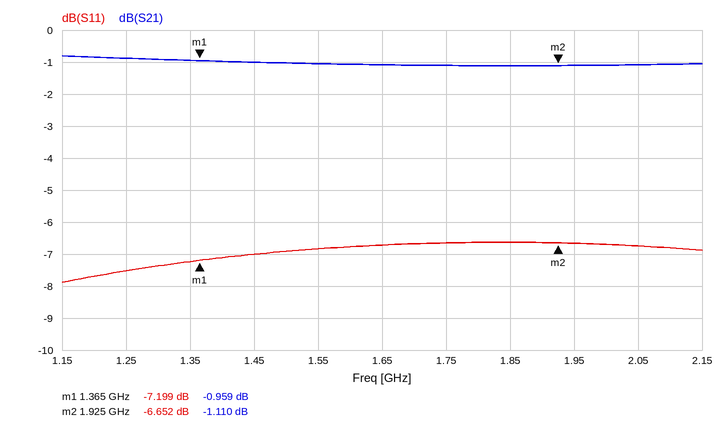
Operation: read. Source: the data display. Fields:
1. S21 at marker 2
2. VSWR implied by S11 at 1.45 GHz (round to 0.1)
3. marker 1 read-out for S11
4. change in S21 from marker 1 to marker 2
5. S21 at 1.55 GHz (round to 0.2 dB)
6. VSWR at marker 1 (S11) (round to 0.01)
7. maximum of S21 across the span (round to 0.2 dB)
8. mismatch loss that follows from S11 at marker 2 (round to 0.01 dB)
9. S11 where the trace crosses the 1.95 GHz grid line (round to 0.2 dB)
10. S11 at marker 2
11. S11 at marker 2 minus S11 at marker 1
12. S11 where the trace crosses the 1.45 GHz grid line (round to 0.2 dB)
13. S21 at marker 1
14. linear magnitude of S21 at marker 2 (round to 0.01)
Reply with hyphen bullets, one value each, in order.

- -1.110 dB
- 2.6
- -7.199 dB
- -0.151 dB
- -1.0 dB
- 2.55
- -0.8 dB
- 1.06 dB
- -6.6 dB
- -6.652 dB
- 0.547 dB
- -7.0 dB
- -0.959 dB
- 0.88
